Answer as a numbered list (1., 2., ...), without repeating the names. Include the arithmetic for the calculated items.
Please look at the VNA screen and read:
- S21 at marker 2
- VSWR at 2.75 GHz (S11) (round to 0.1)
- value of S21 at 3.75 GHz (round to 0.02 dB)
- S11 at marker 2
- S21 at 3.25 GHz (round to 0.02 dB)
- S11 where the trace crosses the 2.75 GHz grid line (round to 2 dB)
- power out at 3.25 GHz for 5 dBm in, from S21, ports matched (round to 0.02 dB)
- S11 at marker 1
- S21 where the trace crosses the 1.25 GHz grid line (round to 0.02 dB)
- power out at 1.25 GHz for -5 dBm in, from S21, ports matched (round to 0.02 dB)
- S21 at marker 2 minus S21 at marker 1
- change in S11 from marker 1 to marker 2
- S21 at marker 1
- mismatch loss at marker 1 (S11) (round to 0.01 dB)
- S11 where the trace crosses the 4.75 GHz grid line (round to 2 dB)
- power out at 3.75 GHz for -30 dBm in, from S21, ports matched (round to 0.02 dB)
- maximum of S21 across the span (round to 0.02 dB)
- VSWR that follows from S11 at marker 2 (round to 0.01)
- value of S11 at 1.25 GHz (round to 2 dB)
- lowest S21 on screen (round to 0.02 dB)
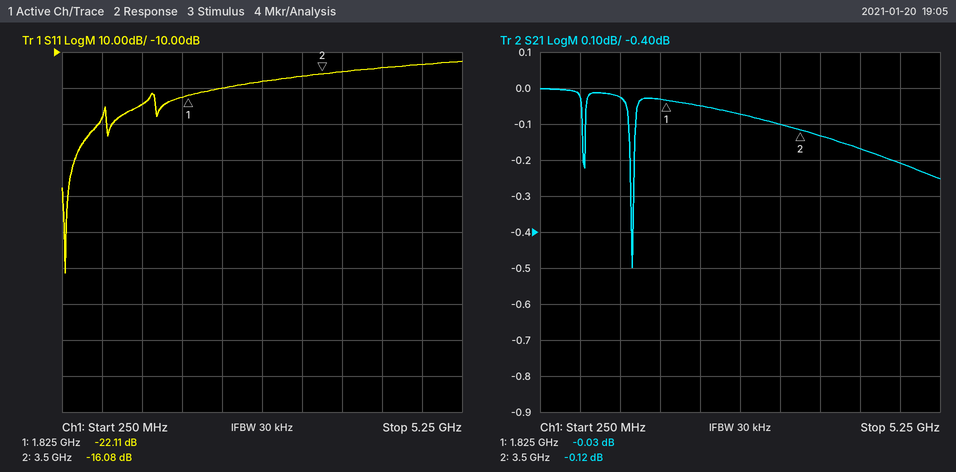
1. -0.12 dB
2. |Γ| = 10^(-18/20) = 0.1259; VSWR = (1 + 0.1259)/(1 − 0.1259) ≈ 1.3
3. -0.14 dB
4. -16.08 dB
5. -0.10 dB
6. -18 dB
7. 5 dBm + (-0.10 dB) = 4.90 dBm
8. -22.11 dB
9. -0.02 dB
10. -5 dBm + (-0.02 dB) = -5.02 dBm
11. -0.12 − (-0.03) = -0.09 dB
12. -16.08 − (-22.11) = 6.03 dB
13. -0.03 dB
14. −10 log10(1 − 10^(-22.11/10)) ≈ 0.03 dB
15. -14 dB
16. -30 dBm + (-0.14 dB) = -30.14 dBm
17. 0.00 dB
18. (1 + 0.1570)/(1 − 0.1570) ≈ 1.37
19. -24 dB
20. -0.50 dB
